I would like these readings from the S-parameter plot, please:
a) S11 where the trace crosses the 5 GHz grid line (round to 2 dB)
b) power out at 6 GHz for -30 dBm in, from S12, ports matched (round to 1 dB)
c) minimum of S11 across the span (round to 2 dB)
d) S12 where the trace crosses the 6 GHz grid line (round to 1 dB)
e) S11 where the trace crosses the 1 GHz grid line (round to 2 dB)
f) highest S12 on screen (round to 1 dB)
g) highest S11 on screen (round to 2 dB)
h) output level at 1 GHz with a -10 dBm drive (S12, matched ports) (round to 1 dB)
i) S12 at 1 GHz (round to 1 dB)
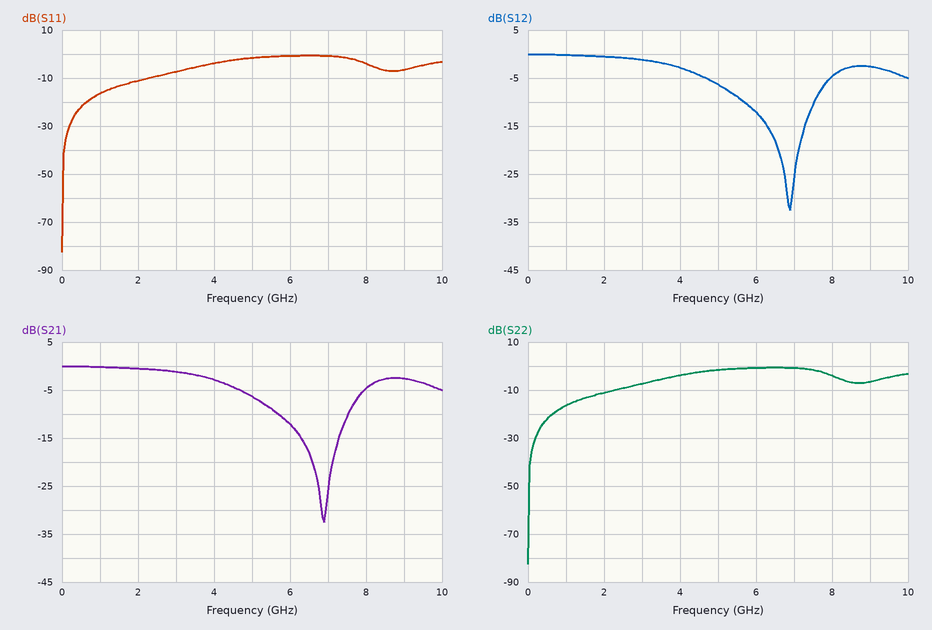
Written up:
-2 dB
-42 dBm
-82 dB
-12 dB
-16 dB
0 dB
0 dB
-10 dBm
0 dB
